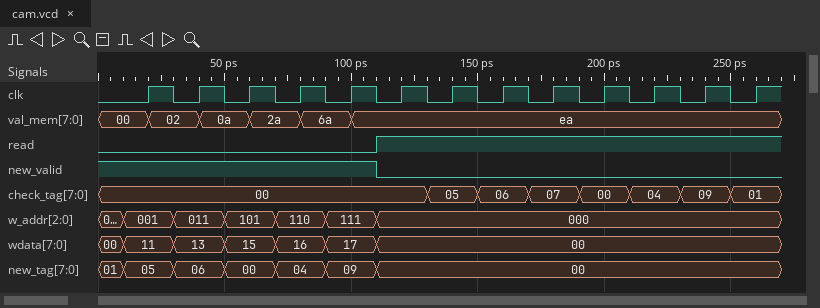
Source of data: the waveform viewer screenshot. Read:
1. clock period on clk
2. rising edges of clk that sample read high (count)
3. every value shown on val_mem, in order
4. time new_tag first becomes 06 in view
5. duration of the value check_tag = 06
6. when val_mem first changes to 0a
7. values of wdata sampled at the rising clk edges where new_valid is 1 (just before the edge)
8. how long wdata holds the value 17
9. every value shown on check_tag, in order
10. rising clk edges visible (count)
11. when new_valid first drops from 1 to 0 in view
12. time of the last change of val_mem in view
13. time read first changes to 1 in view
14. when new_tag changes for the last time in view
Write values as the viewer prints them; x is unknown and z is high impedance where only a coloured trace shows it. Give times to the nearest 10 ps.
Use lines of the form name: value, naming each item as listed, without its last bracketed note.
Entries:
clock period on clk: 20 ps
rising edges of clk that sample read high: 8
every value shown on val_mem, in order: 00, 02, 0a, 2a, 6a, ea
time new_tag first becomes 06 in view: 30 ps
duration of the value check_tag = 06: 20 ps
when val_mem first changes to 0a: 40 ps
values of wdata sampled at the rising clk edges where new_valid is 1: 11, 13, 15, 16, 17
how long wdata holds the value 17: 20 ps
every value shown on check_tag, in order: 00, 05, 06, 07, 00, 04, 09, 01
rising clk edges visible: 13
when new_valid first drops from 1 to 0 in view: 110 ps
time of the last change of val_mem in view: 100 ps
time read first changes to 1 in view: 110 ps
when new_tag changes for the last time in view: 110 ps
